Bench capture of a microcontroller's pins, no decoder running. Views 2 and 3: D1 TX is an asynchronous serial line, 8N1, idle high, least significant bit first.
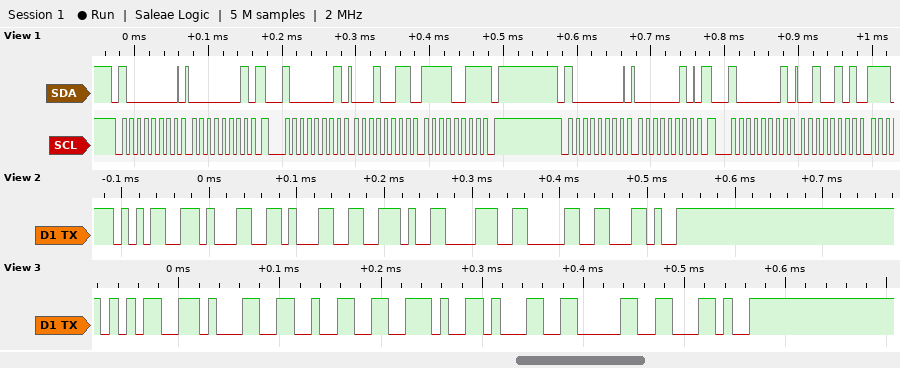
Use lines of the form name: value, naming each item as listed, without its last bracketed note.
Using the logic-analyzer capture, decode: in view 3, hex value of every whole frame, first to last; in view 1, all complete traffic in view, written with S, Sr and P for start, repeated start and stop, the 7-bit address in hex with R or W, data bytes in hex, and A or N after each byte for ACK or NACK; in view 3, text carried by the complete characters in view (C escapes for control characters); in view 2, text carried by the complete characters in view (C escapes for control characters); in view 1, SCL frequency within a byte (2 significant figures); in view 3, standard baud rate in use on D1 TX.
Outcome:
in view 3, hex value of every whole frame, first to last: 0x35 0x31 0x32 0x2E 0x31 0x30 0x2C
in view 1, all complete traffic in view, written with S, Sr and P for start, repeated start and stop, the 7-bit address in hex with R or W, data bytes in hex, and A or N after each byte for ACK or NACK: S 40W A 01 A Sr 40R A 13 A F3 N P S 40W A 02 A Sr 40R A 25 A
in view 3, text carried by the complete characters in view: "512.10,"
in view 2, text carried by the complete characters in view: "511.80,"
in view 1, SCL frequency within a byte: 100 kHz
in view 3, standard baud rate in use on D1 TX: 115200 baud
